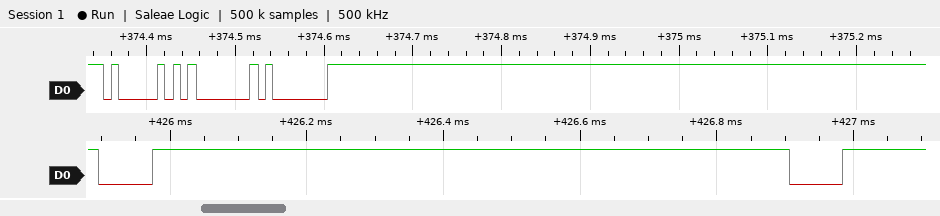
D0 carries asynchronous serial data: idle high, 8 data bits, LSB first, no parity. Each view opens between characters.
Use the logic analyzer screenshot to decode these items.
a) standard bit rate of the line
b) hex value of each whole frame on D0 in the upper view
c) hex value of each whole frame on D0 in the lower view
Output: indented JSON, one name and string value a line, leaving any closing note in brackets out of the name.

{
  "standard bit rate of the line": "115200 baud",
  "hex value of each whole frame on D0 in the upper view": "41, 01, 01",
  "hex value of each whole frame on D0 in the lower view": "00, 00"
}
